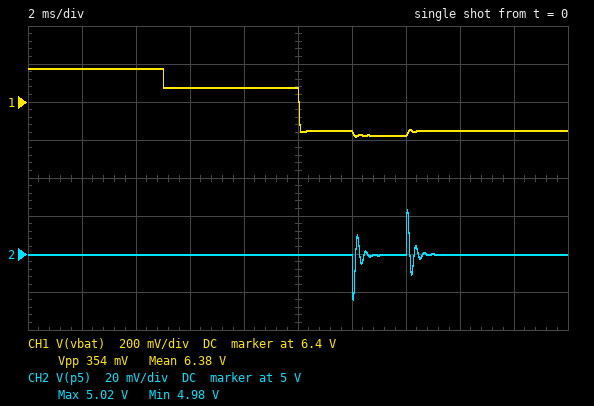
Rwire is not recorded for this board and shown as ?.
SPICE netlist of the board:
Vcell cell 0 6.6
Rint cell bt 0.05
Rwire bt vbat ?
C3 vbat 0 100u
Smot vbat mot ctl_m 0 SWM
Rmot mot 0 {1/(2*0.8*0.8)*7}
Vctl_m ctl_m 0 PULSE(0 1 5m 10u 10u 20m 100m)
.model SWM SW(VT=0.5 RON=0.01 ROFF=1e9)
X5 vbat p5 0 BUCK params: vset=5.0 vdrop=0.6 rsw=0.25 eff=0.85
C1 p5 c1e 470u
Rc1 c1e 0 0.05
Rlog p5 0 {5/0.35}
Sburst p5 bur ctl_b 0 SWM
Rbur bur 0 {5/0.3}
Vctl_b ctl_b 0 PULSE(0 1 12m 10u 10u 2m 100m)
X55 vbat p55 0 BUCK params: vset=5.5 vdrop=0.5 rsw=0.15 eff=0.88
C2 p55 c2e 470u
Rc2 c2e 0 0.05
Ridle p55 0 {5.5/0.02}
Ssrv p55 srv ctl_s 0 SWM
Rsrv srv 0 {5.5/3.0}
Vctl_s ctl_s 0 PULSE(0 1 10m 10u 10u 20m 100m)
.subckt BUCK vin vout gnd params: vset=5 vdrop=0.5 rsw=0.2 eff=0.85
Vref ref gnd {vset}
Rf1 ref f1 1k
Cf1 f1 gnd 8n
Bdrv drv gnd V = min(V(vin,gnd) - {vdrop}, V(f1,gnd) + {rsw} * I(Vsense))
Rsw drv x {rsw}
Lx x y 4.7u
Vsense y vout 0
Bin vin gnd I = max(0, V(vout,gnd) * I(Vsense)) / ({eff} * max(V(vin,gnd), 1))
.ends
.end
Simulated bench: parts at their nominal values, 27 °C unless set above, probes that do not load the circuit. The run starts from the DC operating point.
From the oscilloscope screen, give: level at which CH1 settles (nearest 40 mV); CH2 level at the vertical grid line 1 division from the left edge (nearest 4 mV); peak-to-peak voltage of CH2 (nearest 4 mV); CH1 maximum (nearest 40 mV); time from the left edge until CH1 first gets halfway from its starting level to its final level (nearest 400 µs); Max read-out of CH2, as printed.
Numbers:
6.24 V
5.000 V
48 mV
6.56 V
10.0 ms
5.02 V
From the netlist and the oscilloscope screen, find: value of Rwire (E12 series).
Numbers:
0.033 Ω
